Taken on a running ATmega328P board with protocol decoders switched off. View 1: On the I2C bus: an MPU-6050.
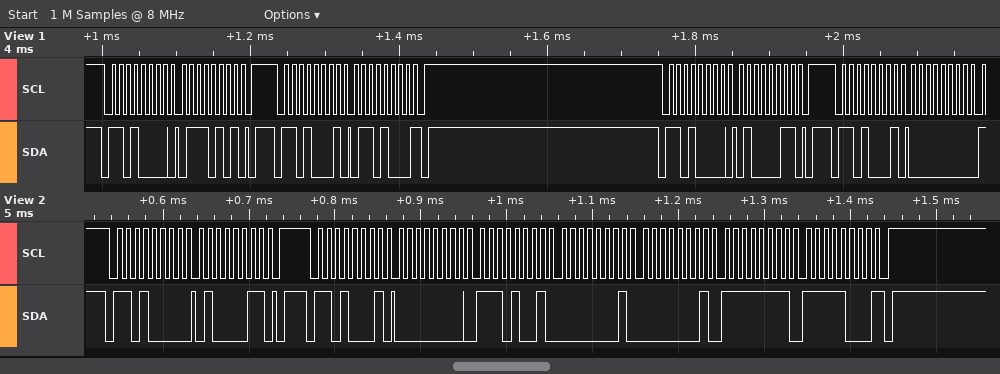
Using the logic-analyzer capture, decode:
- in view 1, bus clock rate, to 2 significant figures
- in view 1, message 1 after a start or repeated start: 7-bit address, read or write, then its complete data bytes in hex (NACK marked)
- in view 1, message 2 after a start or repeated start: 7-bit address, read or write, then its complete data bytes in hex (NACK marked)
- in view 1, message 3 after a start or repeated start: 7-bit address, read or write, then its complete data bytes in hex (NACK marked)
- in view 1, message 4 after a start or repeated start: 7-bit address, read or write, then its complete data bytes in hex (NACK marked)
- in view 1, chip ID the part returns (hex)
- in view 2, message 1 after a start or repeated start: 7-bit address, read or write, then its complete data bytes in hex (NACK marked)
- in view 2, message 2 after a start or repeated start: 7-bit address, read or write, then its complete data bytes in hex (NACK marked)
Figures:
100 kHz
0x68 write: 75
0x68 read: 68 NACK
0x68 write: 43
0x68 read: 00
0x68
0x68 write: 43
0x68 read: 00 E9 01 01 FF F8 NACK
